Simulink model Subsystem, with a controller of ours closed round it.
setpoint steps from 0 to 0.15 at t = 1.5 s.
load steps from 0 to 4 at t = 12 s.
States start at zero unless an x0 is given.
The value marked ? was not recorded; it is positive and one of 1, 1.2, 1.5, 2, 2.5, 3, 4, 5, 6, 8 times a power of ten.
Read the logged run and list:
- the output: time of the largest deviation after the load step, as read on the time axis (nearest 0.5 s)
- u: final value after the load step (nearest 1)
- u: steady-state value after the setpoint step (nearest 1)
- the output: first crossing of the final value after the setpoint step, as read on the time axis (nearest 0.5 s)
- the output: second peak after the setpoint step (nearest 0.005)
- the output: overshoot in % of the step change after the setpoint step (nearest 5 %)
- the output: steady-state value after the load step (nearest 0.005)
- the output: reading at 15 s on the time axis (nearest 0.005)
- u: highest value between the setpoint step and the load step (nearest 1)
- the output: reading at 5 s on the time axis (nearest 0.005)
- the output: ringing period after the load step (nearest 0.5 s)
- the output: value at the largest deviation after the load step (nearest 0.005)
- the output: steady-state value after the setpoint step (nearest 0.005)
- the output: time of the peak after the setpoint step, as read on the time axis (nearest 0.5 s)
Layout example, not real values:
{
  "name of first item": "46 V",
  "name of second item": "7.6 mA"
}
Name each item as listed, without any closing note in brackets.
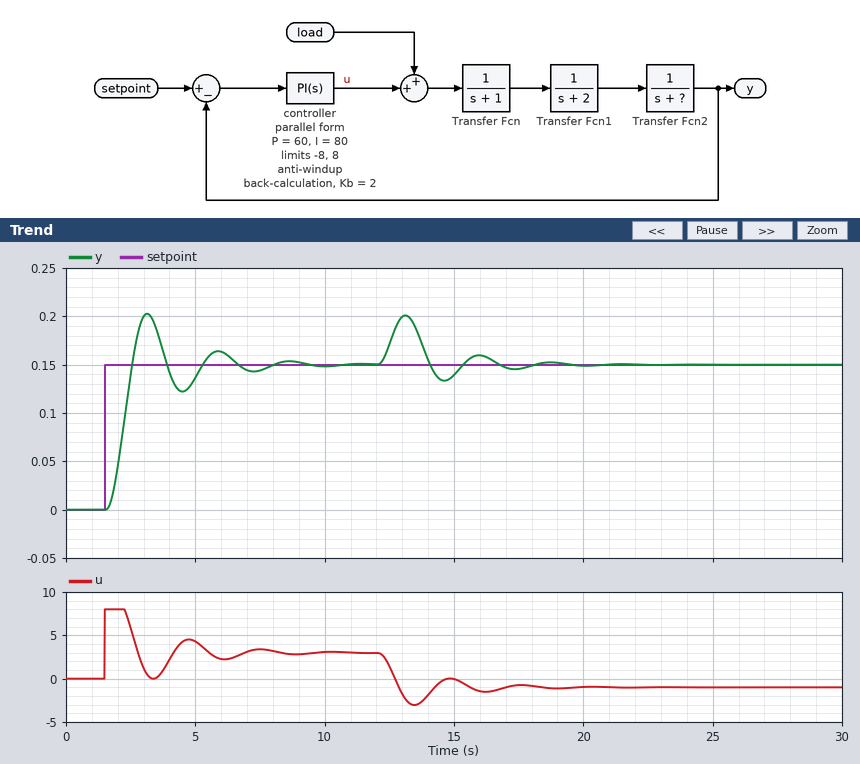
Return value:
{
  "the output: time of the largest deviation after the load step, as read on the time axis": "13.0 s",
  "u: final value after the load step": "-1",
  "u: steady-state value after the setpoint step": "3",
  "the output: first crossing of the final value after the setpoint step, as read on the time axis": "2.5 s",
  "the output: second peak after the setpoint step": "0.165",
  "the output: overshoot in % of the step change after the setpoint step": "35 %",
  "the output: steady-state value after the load step": "0.150",
  "the output: reading at 15 s on the time axis": "0.140",
  "u: highest value between the setpoint step and the load step": "8",
  "the output: reading at 5 s on the time axis": "0.135",
  "the output: ringing period after the load step": "3.0 s",
  "the output: value at the largest deviation after the load step": "0.200",
  "the output: steady-state value after the setpoint step": "0.150",
  "the output: time of the peak after the setpoint step, as read on the time axis": "3.0 s"
}
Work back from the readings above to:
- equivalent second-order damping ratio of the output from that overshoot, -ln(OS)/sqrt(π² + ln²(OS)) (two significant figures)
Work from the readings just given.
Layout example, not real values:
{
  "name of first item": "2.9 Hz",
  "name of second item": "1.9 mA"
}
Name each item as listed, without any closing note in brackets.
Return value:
{
  "equivalent second-order damping ratio of the output from that overshoot, -ln(OS)/sqrt(π² + ln²(OS))": "0.32"
}
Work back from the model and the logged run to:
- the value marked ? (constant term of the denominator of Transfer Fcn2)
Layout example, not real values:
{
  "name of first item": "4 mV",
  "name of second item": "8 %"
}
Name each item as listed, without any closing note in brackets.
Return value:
{
  "the value marked ?": "10"
}
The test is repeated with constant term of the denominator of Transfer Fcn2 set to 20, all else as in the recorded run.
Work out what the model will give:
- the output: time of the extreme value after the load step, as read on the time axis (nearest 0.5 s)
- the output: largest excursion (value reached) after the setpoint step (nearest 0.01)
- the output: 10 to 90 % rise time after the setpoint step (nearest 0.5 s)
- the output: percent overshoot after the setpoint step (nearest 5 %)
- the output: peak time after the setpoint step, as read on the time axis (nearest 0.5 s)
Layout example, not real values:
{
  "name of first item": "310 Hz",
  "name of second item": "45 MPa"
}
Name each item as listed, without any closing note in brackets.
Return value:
{
  "the output: time of the extreme value after the load step, as read on the time axis": "13.5 s",
  "the output: largest excursion (value reached) after the setpoint step": "0.16",
  "the output: 10 to 90 % rise time after the setpoint step": "1.5 s",
  "the output: percent overshoot after the setpoint step": "10 %",
  "the output: peak time after the setpoint step, as read on the time axis": "4.5 s"
}
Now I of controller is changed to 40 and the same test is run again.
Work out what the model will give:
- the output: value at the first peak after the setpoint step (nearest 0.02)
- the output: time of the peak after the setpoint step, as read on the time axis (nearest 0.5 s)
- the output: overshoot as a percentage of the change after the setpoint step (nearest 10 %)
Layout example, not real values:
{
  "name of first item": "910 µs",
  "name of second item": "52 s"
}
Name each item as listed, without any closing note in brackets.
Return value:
{
  "the output: value at the first peak after the setpoint step": "0.18",
  "the output: time of the peak after the setpoint step, as read on the time axis": "3.0 s",
  "the output: overshoot as a percentage of the change after the setpoint step": "20 %"
}
